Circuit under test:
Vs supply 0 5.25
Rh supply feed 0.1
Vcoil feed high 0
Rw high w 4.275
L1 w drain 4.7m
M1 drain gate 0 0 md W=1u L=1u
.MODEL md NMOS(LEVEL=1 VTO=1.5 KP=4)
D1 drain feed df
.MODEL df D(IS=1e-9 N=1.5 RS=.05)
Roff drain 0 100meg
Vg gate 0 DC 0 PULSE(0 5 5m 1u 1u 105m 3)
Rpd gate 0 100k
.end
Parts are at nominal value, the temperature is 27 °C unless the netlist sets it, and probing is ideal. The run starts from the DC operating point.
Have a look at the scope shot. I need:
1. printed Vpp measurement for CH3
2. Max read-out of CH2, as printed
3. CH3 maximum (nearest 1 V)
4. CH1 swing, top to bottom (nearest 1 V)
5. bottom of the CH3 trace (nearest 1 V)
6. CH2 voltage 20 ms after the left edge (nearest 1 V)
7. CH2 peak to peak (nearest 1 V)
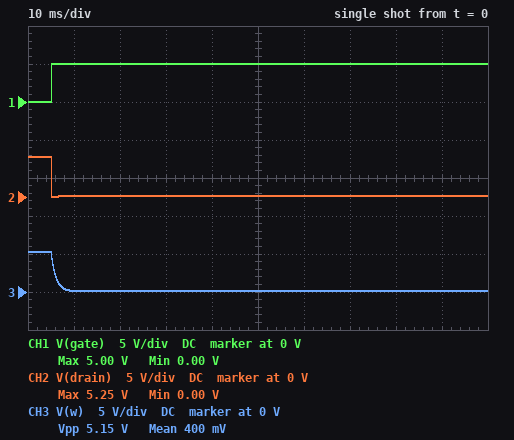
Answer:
5.15 V
5.25 V
5 V
5 V
0 V
0 V
5 V
